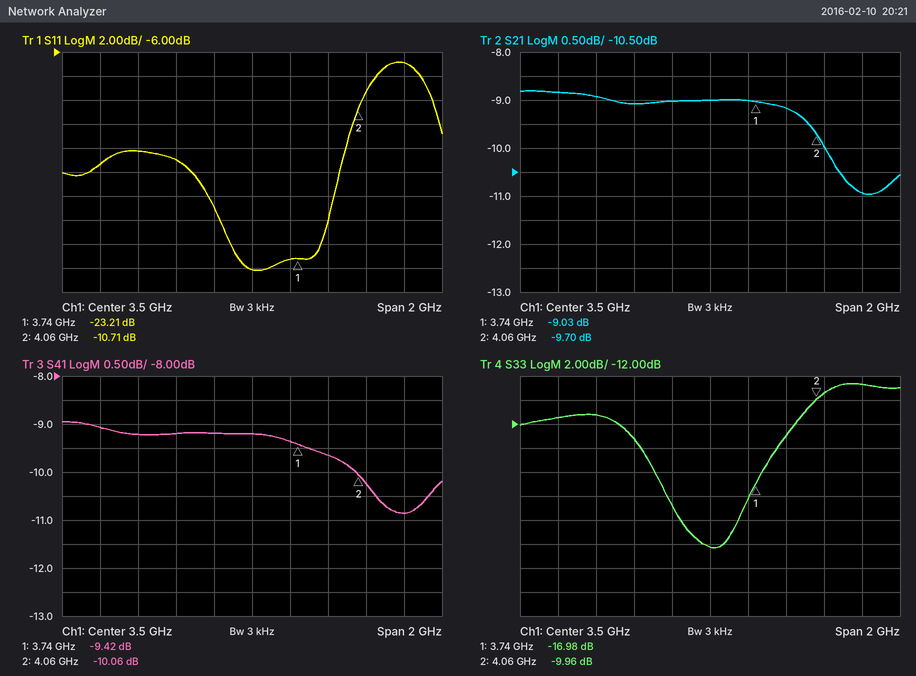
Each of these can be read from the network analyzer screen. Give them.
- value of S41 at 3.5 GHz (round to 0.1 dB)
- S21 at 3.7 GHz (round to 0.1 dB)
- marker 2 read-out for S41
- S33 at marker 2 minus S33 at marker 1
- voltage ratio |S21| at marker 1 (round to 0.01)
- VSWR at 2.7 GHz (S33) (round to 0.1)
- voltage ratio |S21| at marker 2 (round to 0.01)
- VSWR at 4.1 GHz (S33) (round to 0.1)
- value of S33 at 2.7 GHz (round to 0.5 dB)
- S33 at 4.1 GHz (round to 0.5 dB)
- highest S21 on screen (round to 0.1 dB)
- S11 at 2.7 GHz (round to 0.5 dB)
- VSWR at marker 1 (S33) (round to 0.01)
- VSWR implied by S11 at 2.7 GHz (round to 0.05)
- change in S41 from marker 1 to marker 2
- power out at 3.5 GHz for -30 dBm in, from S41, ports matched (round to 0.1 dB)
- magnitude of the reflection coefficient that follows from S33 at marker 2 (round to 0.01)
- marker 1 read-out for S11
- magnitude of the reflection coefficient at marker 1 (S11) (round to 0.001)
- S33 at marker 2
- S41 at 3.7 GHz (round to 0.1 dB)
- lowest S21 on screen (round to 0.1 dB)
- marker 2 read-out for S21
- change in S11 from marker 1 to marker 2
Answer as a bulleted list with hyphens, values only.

- -9.2 dB
- -9.0 dB
- -10.06 dB
- 7.02 dB
- 0.35
- 1.7
- 0.33
- 2.0
- -11.5 dB
- -9.5 dB
- -8.8 dB
- -15.5 dB
- 1.33
- 1.40
- -0.64 dB
- -39.2 dBm
- 0.32
- -23.21 dB
- 0.069
- -9.96 dB
- -9.4 dB
- -11.0 dB
- -9.70 dB
- 12.50 dB
